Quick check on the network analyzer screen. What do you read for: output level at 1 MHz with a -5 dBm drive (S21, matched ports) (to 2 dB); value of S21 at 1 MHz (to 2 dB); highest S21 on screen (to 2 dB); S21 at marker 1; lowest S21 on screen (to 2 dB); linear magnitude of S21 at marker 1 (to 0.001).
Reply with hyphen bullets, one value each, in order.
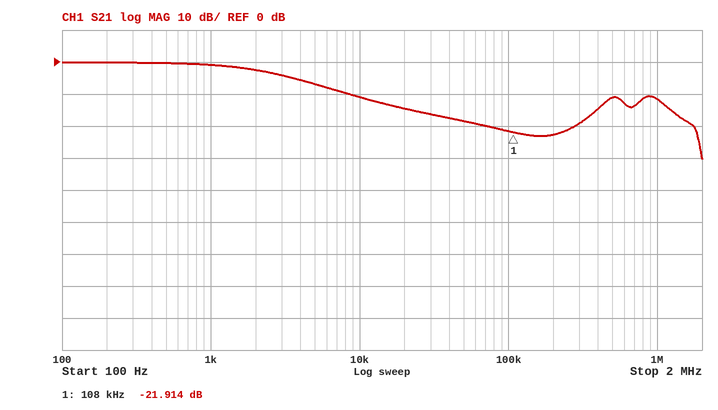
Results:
- -16 dBm
- -12 dB
- 0 dB
- -21.914 dB
- -30 dB
- 0.080
